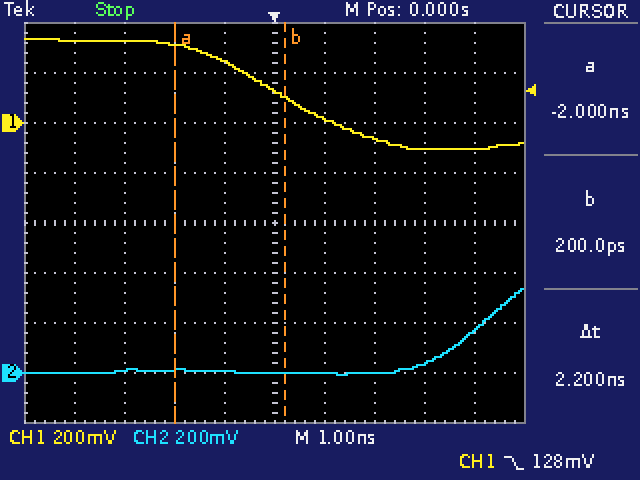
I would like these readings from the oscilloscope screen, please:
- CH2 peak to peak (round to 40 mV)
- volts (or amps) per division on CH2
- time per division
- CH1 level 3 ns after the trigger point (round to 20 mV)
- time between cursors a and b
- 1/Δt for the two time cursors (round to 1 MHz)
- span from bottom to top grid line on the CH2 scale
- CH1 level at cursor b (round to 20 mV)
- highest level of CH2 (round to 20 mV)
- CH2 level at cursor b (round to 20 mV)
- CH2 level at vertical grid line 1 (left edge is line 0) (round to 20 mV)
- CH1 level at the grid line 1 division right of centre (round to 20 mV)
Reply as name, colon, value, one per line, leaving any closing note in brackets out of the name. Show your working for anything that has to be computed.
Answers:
CH2 peak to peak: 360 mV
volts (or amps) per division on CH2: 200 mV
time per division: 1 ns
CH1 level 3 ns after the trigger point: -100 mV
time between cursors a and b: 2.2 ns
1/Δt for the two time cursors: 1 / 2.2 ns ≈ 455 MHz
span from bottom to top grid line on the CH2 scale: 1.6 V
CH1 level at cursor b: 100 mV
highest level of CH2: 340 mV
CH2 level at cursor b: 0 mV
CH2 level at vertical grid line 1 (left edge is line 0): 0 mV
CH1 level at the grid line 1 division right of centre: 20 mV
